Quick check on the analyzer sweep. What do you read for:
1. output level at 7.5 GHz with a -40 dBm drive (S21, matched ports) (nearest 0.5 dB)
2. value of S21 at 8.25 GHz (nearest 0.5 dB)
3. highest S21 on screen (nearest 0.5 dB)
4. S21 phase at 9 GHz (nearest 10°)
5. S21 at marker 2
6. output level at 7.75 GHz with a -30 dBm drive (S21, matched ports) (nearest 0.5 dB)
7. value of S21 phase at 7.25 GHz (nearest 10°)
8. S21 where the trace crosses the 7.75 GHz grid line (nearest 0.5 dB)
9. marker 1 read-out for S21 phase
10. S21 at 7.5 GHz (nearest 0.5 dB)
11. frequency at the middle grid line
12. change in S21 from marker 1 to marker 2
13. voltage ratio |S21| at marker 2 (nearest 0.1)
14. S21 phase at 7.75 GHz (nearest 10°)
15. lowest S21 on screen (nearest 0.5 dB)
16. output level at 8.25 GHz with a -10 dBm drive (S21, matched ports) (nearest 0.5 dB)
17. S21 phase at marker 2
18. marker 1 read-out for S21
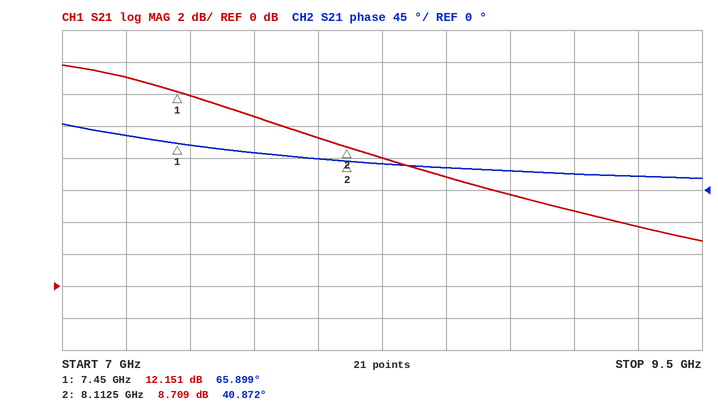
-28.0 dBm
8.0 dB
14.0 dB
20°
8.709 dB
-19.5 dBm
80°
10.5 dB
65.899°
12.0 dB
8.25 GHz
-3.442 dB
2.7
50°
3.0 dB
-2.0 dBm
40.872°
12.151 dB
